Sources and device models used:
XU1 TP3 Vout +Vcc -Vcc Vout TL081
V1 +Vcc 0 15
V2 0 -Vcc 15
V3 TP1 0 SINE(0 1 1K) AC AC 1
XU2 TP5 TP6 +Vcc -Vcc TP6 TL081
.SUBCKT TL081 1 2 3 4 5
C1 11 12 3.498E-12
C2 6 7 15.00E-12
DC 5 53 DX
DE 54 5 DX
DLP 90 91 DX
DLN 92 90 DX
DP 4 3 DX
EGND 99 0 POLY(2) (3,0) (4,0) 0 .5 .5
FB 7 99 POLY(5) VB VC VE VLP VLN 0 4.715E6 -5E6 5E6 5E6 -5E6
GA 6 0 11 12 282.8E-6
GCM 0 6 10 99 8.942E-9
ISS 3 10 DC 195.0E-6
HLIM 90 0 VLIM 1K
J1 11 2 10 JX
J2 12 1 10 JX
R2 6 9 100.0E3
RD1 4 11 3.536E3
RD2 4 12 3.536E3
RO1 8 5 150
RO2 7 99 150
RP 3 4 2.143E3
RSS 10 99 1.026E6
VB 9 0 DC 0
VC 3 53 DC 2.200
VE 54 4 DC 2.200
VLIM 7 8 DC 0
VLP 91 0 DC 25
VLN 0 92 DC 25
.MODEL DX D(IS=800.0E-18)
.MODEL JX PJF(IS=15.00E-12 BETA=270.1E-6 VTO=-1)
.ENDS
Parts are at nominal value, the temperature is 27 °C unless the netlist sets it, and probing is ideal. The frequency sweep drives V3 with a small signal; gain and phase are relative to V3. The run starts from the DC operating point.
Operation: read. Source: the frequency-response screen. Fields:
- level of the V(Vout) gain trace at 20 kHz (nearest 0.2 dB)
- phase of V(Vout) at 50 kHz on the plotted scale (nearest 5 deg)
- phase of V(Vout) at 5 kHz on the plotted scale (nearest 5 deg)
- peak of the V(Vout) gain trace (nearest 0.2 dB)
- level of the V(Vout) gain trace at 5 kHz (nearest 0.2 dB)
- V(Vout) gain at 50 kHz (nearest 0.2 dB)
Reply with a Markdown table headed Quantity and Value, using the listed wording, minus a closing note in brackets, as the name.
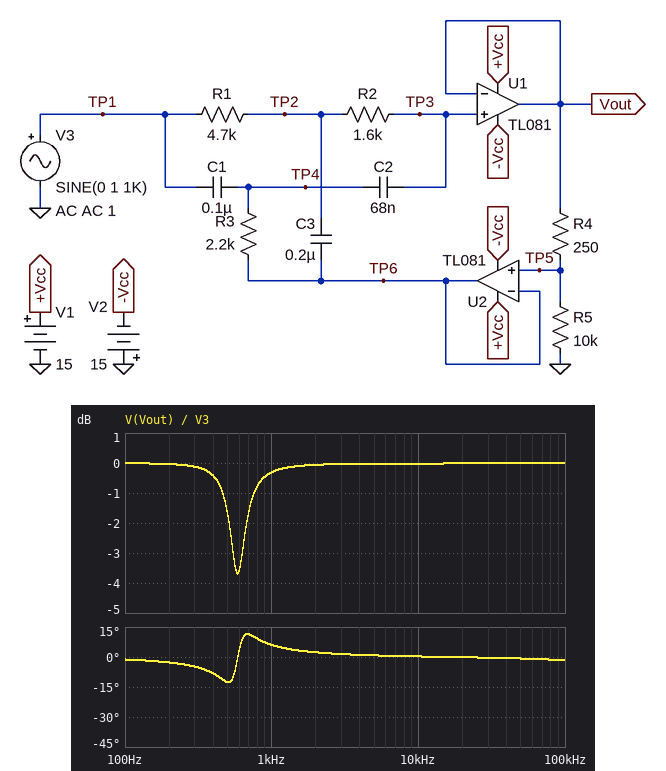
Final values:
| Quantity | Value |
|---|---|
| level of the V(Vout) gain trace at 20 kHz | 0 dB |
| phase of V(Vout) at 50 kHz on the plotted scale | 0 deg |
| phase of V(Vout) at 5 kHz on the plotted scale | 0 deg |
| peak of the V(Vout) gain trace | 0 dB |
| level of the V(Vout) gain trace at 5 kHz | 0 dB |
| V(Vout) gain at 50 kHz | 0 dB |
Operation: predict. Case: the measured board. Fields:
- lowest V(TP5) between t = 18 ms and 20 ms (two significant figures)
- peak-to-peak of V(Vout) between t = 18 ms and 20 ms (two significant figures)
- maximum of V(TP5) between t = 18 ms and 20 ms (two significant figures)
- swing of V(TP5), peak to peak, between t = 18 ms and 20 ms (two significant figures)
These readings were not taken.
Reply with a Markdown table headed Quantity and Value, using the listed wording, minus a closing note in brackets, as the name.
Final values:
| Quantity | Value |
|---|---|
| lowest V(TP5) between t = 18 ms and 20 ms | -940 mV |
| peak-to-peak of V(Vout) between t = 18 ms and 20 ms | 1.9 V |
| maximum of V(TP5) between t = 18 ms and 20 ms | 940 mV |
| swing of V(TP5), peak to peak, between t = 18 ms and 20 ms | 1.9 V |
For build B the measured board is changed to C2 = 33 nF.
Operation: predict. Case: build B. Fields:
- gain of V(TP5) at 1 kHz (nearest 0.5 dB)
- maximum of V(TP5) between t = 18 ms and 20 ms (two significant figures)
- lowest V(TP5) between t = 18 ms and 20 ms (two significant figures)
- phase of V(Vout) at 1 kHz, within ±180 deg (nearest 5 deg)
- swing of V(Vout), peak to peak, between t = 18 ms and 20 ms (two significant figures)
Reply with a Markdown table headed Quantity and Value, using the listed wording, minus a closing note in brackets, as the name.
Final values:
| Quantity | Value |
|---|---|
| gain of V(TP5) at 1 kHz | -1.0 dB |
| maximum of V(TP5) between t = 18 ms and 20 ms | 870 mV |
| lowest V(TP5) between t = 18 ms and 20 ms | -870 mV |
| phase of V(Vout) at 1 kHz, within ±180 deg | 15 deg |
| swing of V(Vout), peak to peak, between t = 18 ms and 20 ms | 1.8 V |
